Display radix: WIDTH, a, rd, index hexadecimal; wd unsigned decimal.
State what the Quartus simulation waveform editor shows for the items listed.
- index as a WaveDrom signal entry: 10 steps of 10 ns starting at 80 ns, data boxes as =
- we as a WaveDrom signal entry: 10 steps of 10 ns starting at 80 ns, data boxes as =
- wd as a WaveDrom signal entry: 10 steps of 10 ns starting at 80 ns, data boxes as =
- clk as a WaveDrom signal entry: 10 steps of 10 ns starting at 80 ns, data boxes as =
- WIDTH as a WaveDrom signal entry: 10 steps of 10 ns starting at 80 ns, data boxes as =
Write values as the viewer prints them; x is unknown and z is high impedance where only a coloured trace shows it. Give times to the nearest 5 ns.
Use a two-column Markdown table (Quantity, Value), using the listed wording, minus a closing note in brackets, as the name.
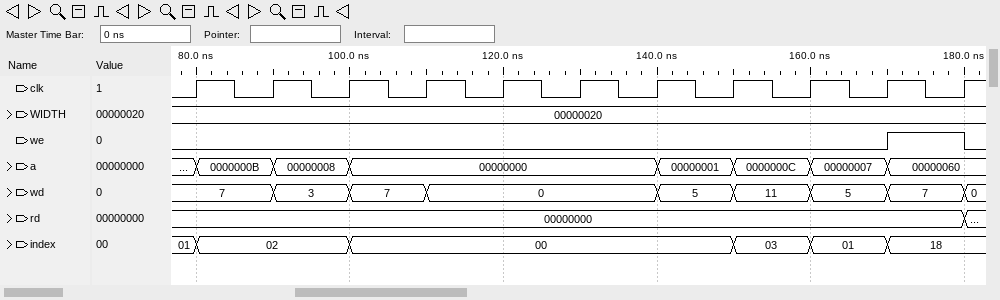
| Quantity | Value |
|---|---|
| index as a WaveDrom signal entry: 10 steps of 10 ns starting at 80 ns, data boxes as = | {name: 'index', wave: '=.=....===', data: '02 00 03 01 18'} |
| we as a WaveDrom signal entry: 10 steps of 10 ns starting at 80 ns, data boxes as = | {name: 'we', wave: '0........1'} |
| wd as a WaveDrom signal entry: 10 steps of 10 ns starting at 80 ns, data boxes as = | {name: 'wd', wave: '====..====', data: '7 3 7 0 5 11 5 7'} |
| clk as a WaveDrom signal entry: 10 steps of 10 ns starting at 80 ns, data boxes as = | {name: 'clk', wave: 'p.........'} |
| WIDTH as a WaveDrom signal entry: 10 steps of 10 ns starting at 80 ns, data boxes as = | {name: 'WIDTH', wave: '=.........', data: '00000020'} |
